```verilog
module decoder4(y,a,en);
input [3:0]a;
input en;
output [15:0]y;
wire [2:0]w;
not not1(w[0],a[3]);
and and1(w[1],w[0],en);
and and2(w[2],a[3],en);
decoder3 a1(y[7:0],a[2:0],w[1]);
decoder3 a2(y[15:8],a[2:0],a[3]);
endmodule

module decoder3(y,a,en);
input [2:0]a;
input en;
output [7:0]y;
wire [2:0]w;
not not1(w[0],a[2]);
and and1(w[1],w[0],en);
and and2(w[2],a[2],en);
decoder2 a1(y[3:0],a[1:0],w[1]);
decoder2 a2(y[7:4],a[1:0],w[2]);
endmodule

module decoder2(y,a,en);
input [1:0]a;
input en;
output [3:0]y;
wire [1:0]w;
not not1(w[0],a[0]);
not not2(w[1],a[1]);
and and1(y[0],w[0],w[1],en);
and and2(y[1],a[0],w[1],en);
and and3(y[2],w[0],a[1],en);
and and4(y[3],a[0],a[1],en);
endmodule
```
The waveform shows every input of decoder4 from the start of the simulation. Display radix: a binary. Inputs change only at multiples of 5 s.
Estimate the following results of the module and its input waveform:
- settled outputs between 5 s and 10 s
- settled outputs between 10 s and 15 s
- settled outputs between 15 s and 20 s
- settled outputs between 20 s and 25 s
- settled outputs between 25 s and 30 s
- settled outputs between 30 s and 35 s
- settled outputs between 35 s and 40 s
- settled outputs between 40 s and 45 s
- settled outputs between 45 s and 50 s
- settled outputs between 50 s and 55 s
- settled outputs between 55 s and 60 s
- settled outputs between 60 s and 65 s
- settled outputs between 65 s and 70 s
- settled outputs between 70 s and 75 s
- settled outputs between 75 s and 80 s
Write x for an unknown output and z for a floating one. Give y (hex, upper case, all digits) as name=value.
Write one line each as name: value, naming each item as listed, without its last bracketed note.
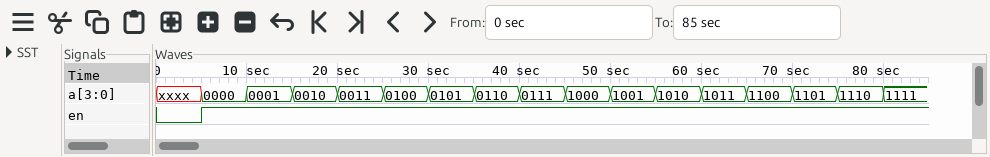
settled outputs between 5 s and 10 s: y=0001
settled outputs between 10 s and 15 s: y=0002
settled outputs between 15 s and 20 s: y=0004
settled outputs between 20 s and 25 s: y=0008
settled outputs between 25 s and 30 s: y=0010
settled outputs between 30 s and 35 s: y=0020
settled outputs between 35 s and 40 s: y=0040
settled outputs between 40 s and 45 s: y=0080
settled outputs between 45 s and 50 s: y=0100
settled outputs between 50 s and 55 s: y=0200
settled outputs between 55 s and 60 s: y=0400
settled outputs between 60 s and 65 s: y=0800
settled outputs between 65 s and 70 s: y=1000
settled outputs between 70 s and 75 s: y=2000
settled outputs between 75 s and 80 s: y=4000
